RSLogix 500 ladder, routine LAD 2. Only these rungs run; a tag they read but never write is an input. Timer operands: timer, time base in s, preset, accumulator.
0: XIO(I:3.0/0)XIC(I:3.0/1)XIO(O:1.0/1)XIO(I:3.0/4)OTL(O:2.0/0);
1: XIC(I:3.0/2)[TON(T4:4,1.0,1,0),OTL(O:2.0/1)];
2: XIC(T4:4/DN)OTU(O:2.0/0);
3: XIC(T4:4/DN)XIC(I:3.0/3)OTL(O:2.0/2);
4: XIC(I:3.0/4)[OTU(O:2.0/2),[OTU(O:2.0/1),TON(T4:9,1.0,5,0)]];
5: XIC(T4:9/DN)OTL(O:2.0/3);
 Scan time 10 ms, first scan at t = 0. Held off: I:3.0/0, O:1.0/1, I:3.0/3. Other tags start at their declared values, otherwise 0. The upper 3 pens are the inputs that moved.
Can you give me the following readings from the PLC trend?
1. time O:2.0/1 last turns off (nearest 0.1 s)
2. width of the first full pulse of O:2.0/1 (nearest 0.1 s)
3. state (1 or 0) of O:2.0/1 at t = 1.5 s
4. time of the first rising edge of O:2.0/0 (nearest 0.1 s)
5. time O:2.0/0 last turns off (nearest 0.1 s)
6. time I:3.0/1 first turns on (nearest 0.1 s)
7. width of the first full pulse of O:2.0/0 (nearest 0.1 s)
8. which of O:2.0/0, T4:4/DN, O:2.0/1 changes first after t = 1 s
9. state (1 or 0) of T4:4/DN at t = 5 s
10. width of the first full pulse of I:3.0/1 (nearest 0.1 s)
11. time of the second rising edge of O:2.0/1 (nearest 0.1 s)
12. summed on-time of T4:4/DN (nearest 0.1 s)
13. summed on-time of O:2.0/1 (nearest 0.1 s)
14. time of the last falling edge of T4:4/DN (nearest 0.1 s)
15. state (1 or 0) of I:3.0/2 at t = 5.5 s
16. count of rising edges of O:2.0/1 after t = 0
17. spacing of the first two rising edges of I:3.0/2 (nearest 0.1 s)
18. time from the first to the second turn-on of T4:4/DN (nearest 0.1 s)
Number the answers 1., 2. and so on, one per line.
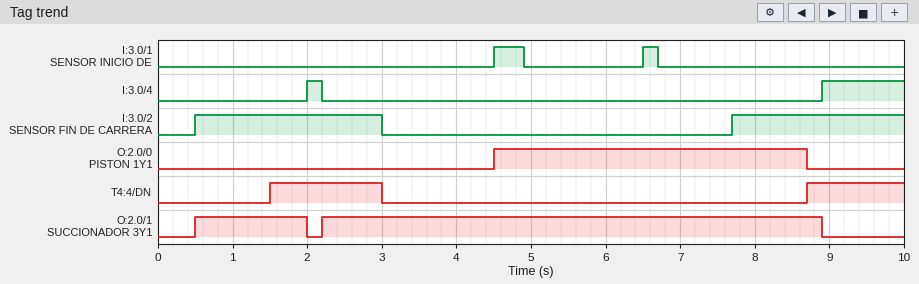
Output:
1. 8.9 s
2. 1.5 s
3. 1
4. 4.5 s
5. 8.7 s
6. 4.5 s
7. 4.2 s
8. T4:4/DN
9. 0
10. 0.4 s
11. 2.2 s
12. 2.8 s
13. 8.2 s
14. 3.0 s
15. 0
16. 2
17. 7.2 s
18. 7.2 s
